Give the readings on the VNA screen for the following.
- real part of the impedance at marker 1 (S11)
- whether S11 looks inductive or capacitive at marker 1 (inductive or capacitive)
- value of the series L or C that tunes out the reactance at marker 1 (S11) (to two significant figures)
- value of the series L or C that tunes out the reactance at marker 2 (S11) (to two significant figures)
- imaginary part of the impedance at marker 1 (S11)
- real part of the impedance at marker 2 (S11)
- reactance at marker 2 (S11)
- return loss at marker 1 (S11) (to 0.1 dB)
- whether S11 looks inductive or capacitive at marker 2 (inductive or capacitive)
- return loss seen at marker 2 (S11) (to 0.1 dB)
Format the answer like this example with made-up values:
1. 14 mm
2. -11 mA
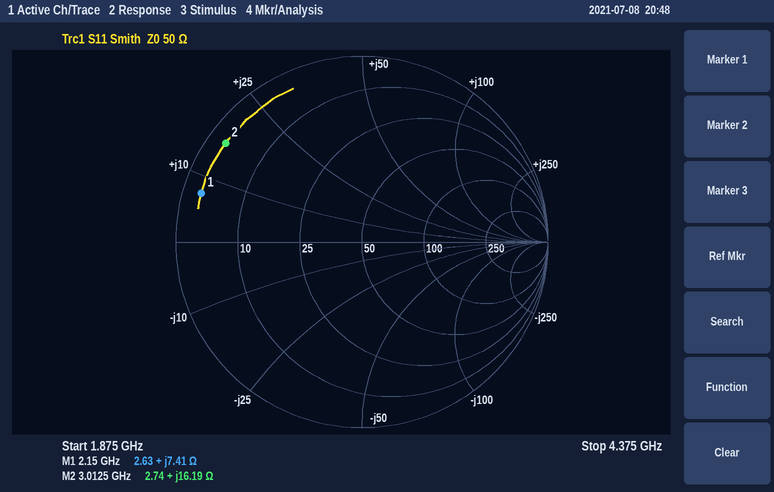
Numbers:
1. 2.63 Ω
2. inductive
3. 10.0 pF
4. 3.3 pF
5. +7.41 Ω
6. 2.74 Ω
7. +16.19 Ω
8. 0.9 dB
9. inductive
10. 0.9 dB
